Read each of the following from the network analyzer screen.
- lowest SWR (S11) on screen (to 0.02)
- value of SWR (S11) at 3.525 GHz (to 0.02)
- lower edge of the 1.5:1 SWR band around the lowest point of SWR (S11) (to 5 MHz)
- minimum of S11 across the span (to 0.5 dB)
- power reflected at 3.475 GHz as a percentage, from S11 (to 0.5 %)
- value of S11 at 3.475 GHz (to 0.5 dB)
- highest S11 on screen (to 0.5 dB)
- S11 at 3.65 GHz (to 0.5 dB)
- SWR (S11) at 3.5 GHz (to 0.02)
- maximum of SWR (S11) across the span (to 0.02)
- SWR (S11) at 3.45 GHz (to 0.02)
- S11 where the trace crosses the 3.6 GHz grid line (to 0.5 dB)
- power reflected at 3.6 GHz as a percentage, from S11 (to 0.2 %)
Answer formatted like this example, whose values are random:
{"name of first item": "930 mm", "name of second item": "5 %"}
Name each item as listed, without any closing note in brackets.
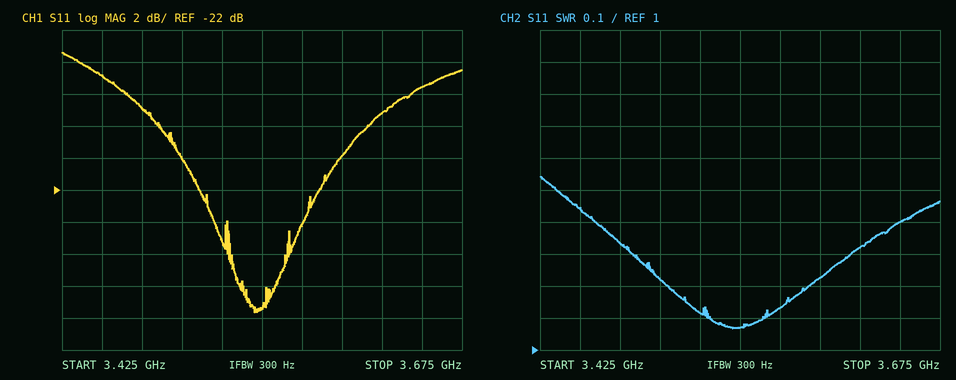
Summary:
{"lowest SWR (S11) on screen": "1.06", "value of SWR (S11) at 3.525 GHz": "1.12", "lower edge of the 1.5:1 SWR band around the lowest point of SWR (S11)": "3.435 GHz", "minimum of S11 across the span": "-29.5 dB", "power reflected at 3.475 GHz as a percentage, from S11": "2.0 %", "value of S11 at 3.475 GHz": "-17.0 dB", "highest S11 on screen": "-13.5 dB", "S11 at 3.65 GHz": "-15.5 dB", "SWR (S11) at 3.5 GHz": "1.22", "maximum of SWR (S11) across the span": "1.54", "SWR (S11) at 3.45 GHz": "1.44", "S11 where the trace crosses the 3.6 GHz grid line": "-20.0 dB", "power reflected at 3.6 GHz as a percentage, from S11": "1.0 %"}
